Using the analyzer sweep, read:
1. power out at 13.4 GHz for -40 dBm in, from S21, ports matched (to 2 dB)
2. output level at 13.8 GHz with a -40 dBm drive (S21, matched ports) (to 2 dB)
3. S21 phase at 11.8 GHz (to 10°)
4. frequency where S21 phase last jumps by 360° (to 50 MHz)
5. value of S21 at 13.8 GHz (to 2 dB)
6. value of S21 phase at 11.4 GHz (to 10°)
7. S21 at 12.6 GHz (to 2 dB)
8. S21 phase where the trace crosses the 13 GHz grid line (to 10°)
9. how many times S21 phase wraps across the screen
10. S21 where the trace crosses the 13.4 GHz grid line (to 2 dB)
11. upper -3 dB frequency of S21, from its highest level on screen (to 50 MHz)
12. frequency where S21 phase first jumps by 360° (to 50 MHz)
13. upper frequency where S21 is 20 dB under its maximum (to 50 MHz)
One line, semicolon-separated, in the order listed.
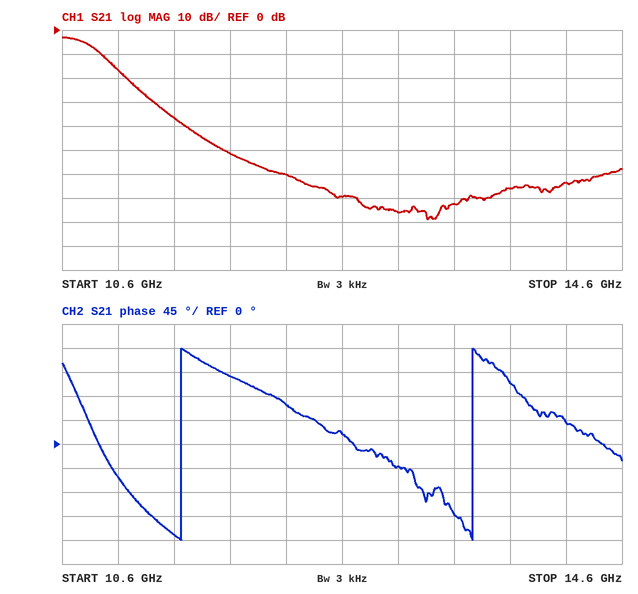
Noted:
-112 dBm; -106 dBm; 130°; 13.55 GHz; -66 dB; -170°; -70 dB; -40°; 2; -72 dB; 10.80 GHz; 11.45 GHz; 11.10 GHz
